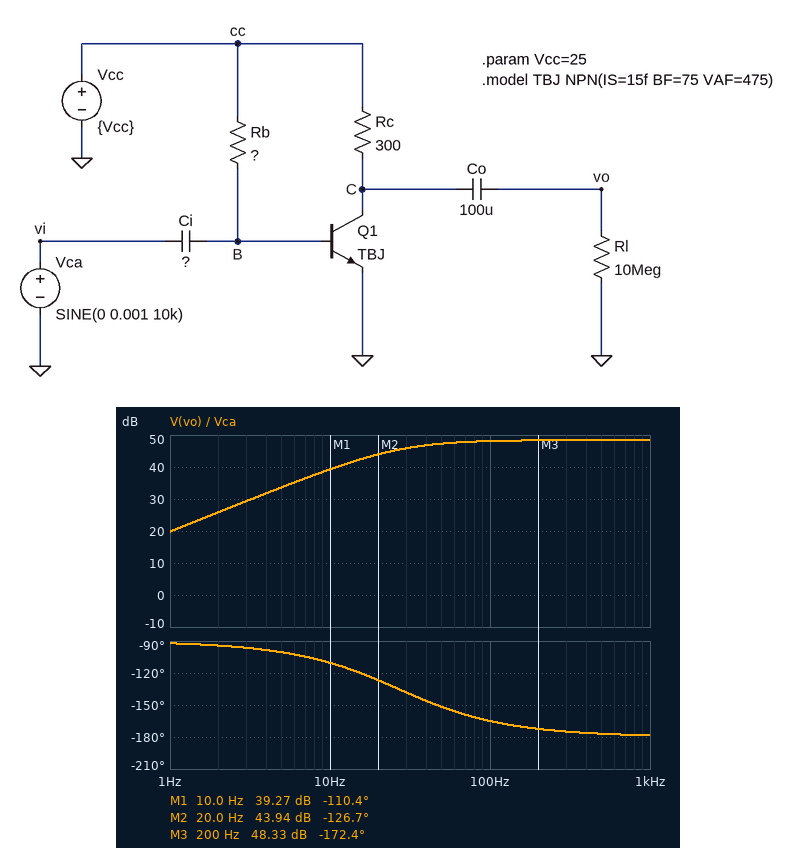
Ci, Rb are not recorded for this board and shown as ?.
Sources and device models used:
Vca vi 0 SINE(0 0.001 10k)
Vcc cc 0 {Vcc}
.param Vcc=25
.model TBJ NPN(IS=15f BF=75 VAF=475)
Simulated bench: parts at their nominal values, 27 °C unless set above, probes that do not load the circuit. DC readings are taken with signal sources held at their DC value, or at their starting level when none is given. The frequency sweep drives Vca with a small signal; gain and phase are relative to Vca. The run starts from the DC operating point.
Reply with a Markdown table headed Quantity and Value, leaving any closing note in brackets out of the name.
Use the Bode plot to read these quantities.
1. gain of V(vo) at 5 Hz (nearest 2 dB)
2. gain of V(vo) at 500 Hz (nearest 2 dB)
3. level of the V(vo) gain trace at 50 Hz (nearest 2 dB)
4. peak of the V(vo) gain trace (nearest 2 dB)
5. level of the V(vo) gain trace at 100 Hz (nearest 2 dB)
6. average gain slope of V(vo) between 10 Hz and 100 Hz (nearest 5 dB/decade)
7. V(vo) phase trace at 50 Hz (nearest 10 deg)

| Quantity | Value |
|---|---|
| gain of V(vo) at 5 Hz | 34 dB |
| gain of V(vo) at 500 Hz | 48 dB |
| level of the V(vo) gain trace at 50 Hz | 48 dB |
| peak of the V(vo) gain trace | 48 dB |
| level of the V(vo) gain trace at 100 Hz | 48 dB |
| average gain slope of V(vo) between 10 Hz and 100 Hz | 10 dB/decade |
| V(vo) phase trace at 50 Hz | -150 deg |
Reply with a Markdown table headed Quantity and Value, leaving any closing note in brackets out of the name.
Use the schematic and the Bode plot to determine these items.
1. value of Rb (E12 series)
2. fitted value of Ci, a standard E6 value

| Quantity | Value |
|---|---|
| value of Rb | 82 kΩ |
| fitted value of Ci, a standard E6 value | 68 µF |
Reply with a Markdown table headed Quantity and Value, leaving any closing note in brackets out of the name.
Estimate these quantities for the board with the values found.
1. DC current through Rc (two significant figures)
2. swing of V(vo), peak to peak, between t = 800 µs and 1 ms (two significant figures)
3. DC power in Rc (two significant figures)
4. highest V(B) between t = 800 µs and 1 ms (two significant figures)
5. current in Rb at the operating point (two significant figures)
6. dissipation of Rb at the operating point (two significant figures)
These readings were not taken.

| Quantity | Value |
|---|---|
| DC current through Rc | 23 mA |
| swing of V(vo), peak to peak, between t = 800 µs and 1 ms | 530 mV |
| DC power in Rc | 160 mW |
| highest V(B) between t = 800 µs and 1 ms | 730 mV |
| current in Rb at the operating point | 300 µA |
| dissipation of Rb at the operating point | 7.2 mW |
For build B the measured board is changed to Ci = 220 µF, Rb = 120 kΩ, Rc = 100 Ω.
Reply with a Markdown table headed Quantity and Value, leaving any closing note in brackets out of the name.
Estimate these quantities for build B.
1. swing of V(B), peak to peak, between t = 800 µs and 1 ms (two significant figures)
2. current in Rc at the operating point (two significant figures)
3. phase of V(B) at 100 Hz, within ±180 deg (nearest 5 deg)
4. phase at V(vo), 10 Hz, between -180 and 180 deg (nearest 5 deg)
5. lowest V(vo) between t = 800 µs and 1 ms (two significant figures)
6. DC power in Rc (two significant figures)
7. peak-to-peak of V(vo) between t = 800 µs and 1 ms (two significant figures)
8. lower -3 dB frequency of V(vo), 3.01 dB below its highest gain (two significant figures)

| Quantity | Value |
|---|---|
| swing of V(B), peak to peak, between t = 800 µs and 1 ms | 2.0 mV |
| current in Rc at the operating point | 16 mA |
| phase of V(B) at 100 Hz, within ±180 deg | 5 deg |
| phase at V(vo), 10 Hz, between -180 and 180 deg | -150 deg |
| lowest V(vo) between t = 800 µs and 1 ms | -62 mV |
| DC power in Rc | 25 mW |
| peak-to-peak of V(vo) between t = 800 µs and 1 ms | 120 mV |
| lower -3 dB frequency of V(vo), 3.01 dB below its highest gain | 5.7 Hz |
